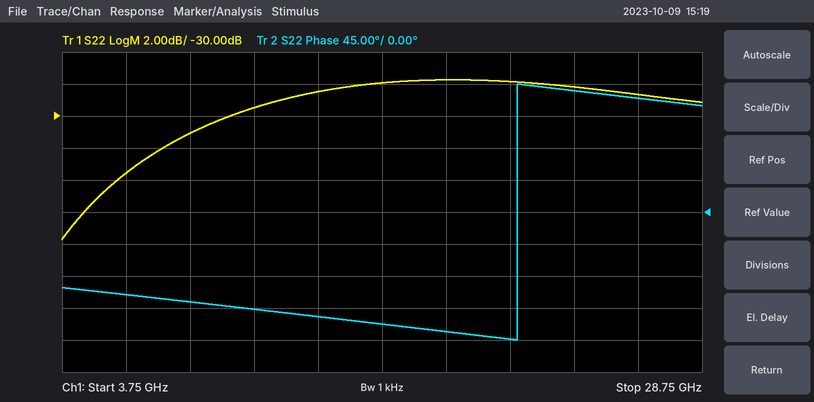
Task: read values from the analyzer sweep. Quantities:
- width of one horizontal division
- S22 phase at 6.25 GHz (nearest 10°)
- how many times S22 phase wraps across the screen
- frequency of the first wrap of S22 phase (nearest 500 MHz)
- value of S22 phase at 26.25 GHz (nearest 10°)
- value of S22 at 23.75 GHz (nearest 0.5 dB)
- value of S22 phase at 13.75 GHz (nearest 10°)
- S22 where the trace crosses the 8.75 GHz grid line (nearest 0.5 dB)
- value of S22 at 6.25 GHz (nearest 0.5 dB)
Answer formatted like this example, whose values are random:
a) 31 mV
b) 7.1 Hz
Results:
a) 2.5 GHz
b) -120°
c) 1
d) 21.5 GHz
e) 160°
f) -28.0 dB
g) -150°
h) -31.0 dB
i) -33.5 dB
